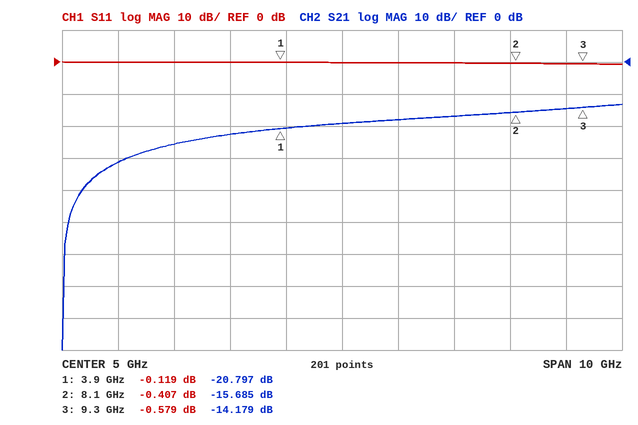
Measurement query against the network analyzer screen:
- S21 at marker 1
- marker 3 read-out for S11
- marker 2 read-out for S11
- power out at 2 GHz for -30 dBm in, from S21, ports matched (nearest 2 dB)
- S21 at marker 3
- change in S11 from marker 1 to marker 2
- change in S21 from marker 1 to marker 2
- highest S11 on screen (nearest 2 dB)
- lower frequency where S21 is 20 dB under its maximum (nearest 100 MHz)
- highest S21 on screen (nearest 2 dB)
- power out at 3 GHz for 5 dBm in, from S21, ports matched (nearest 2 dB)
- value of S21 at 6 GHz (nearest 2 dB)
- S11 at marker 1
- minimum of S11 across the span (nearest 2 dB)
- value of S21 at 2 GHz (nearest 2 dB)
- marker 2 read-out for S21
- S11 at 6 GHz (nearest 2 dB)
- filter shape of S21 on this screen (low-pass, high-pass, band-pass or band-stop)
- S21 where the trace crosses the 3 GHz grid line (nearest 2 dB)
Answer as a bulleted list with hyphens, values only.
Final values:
- -20.797 dB
- -0.579 dB
- -0.407 dB
- -56 dBm
- -14.179 dB
- -0.288 dB
- 5.112 dB
- 0 dB
- 800 MHz
- -14 dB
- -18 dBm
- -18 dB
- -0.119 dB
- 0 dB
- -26 dB
- -15.685 dB
- 0 dB
- high-pass
- -22 dB
